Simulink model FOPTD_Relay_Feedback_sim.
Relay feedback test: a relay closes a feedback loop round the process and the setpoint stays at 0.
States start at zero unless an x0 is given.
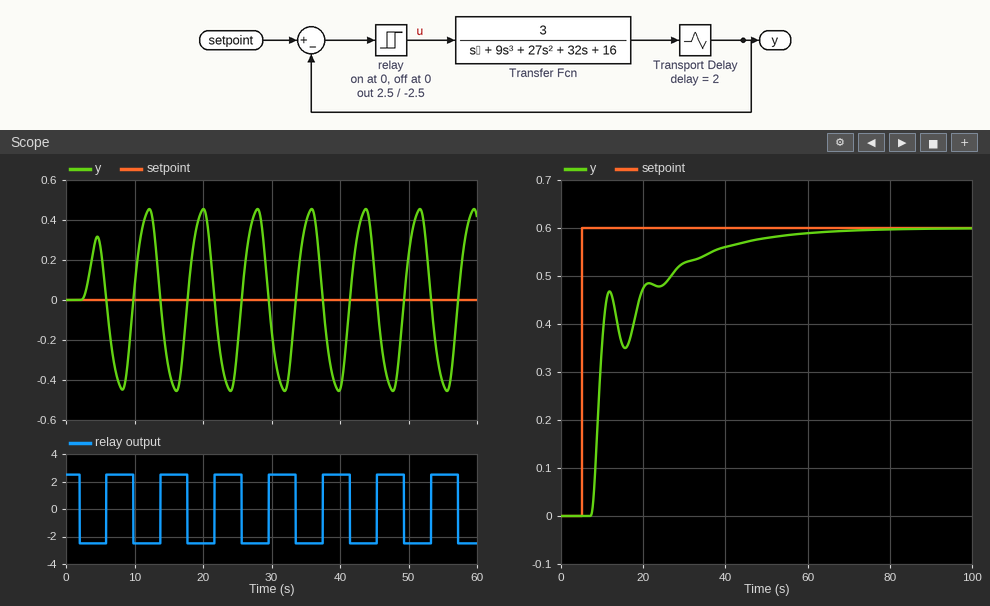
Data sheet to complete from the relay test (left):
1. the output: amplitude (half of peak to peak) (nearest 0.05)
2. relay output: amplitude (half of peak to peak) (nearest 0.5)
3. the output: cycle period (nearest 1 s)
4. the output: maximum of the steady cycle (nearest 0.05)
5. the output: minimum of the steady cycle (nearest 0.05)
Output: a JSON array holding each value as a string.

["0.45", "2.5", "8 s", "0.45", "-0.45"]
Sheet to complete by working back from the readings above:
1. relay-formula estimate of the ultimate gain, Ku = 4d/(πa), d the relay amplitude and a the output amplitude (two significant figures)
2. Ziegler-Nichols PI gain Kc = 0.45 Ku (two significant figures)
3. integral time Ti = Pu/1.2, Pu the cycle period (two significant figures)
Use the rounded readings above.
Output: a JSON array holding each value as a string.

["7.1", "3.2", "6.7 s"]
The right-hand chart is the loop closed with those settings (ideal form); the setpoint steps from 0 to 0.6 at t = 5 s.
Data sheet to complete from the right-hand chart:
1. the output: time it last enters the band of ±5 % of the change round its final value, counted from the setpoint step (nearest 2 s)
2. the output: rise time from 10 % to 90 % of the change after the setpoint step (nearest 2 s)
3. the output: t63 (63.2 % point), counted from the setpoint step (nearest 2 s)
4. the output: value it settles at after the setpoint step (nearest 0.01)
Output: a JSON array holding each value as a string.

["40 s", "26 s", "6 s", "0.60"]
